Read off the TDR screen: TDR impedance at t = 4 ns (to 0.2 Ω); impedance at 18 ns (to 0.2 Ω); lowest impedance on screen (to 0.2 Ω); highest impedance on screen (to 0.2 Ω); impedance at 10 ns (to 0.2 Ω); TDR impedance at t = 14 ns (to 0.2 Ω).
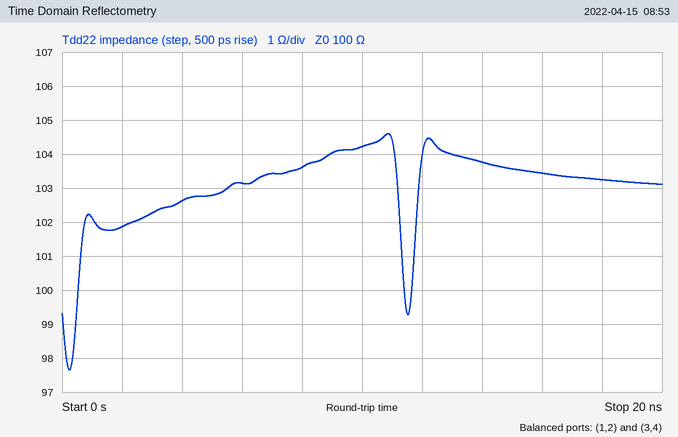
102.6 Ω
103.2 Ω
97.6 Ω
104.6 Ω
104.2 Ω
103.8 Ω
